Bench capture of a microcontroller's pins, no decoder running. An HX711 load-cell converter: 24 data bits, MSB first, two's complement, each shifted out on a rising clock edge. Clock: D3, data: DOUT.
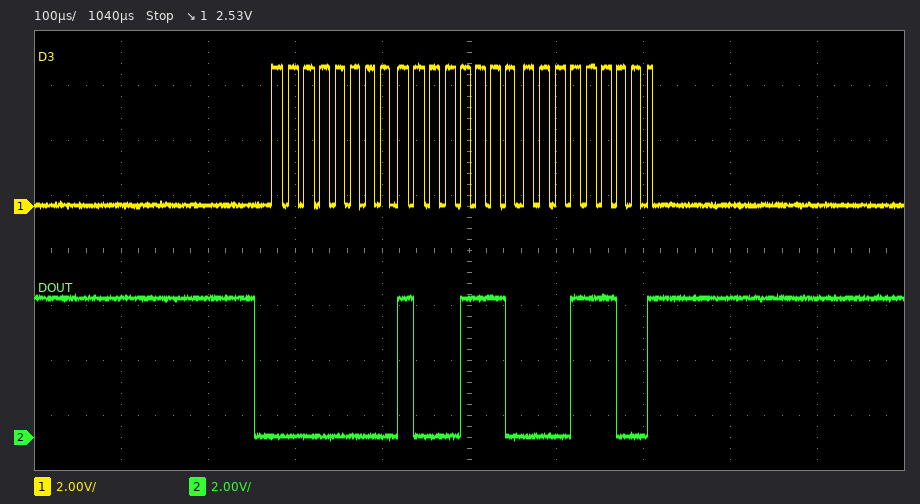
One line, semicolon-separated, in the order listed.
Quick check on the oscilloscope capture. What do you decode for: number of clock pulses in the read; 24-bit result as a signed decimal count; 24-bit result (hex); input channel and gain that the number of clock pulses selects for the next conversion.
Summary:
25; 36380; 0x008E1C; channel A, gain 128
